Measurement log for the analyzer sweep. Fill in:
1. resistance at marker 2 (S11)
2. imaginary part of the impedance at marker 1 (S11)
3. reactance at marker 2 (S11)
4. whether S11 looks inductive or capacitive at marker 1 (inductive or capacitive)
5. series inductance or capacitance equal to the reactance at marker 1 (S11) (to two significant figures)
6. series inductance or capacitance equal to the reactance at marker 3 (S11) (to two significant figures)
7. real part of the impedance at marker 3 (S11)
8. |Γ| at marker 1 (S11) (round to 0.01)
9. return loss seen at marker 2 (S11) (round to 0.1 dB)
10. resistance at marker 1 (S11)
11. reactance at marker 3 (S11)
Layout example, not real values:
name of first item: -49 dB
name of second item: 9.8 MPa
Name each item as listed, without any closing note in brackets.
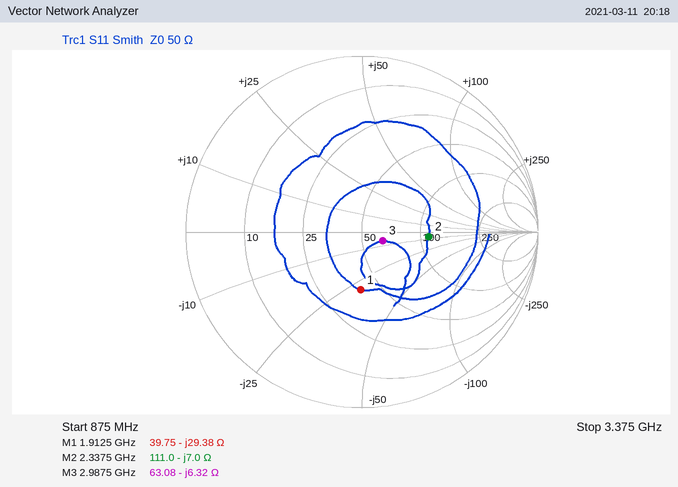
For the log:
resistance at marker 2: 111.0 Ω
imaginary part of the impedance at marker 1: -29.38 Ω
reactance at marker 2: -7.0 Ω
whether S11 looks inductive or capacitive at marker 1: capacitive
series inductance or capacitance equal to the reactance at marker 1 (S11): 2.8 pF
series inductance or capacitance equal to the reactance at marker 3 (S11): 8.4 pF
real part of the impedance at marker 3: 63.08 Ω
|Γ| at marker 1 (S11): 0.33
return loss seen at marker 2 (S11): 8.4 dB
resistance at marker 1: 39.75 Ω
reactance at marker 3: -6.32 Ω
